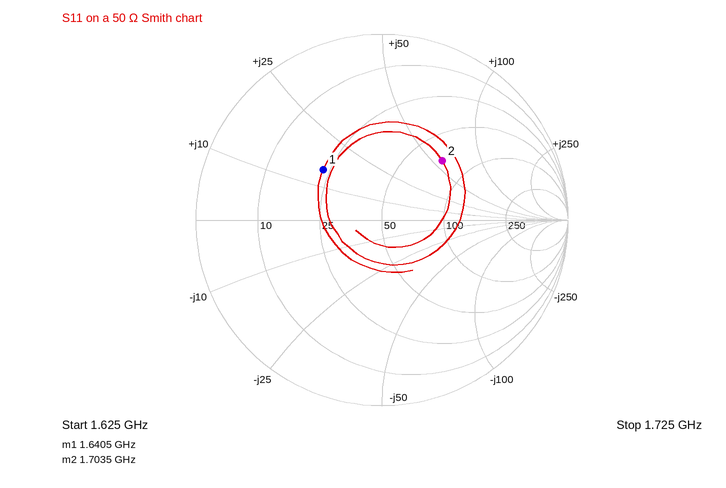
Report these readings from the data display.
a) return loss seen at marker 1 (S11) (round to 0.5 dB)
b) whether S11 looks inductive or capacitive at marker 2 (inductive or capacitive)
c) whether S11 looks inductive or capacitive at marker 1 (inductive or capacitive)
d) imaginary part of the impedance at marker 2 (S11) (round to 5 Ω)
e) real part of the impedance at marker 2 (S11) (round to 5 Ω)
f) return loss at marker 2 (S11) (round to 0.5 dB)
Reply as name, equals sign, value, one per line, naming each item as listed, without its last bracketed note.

return loss seen at marker 1 (S11) = 7.5 dB
whether S11 looks inductive or capacitive at marker 2 = inductive
whether S11 looks inductive or capacitive at marker 1 = inductive
imaginary part of the impedance at marker 2 (S11) = +55 Ω
real part of the impedance at marker 2 (S11) = 70 Ω
return loss at marker 2 (S11) = 7.0 dB
